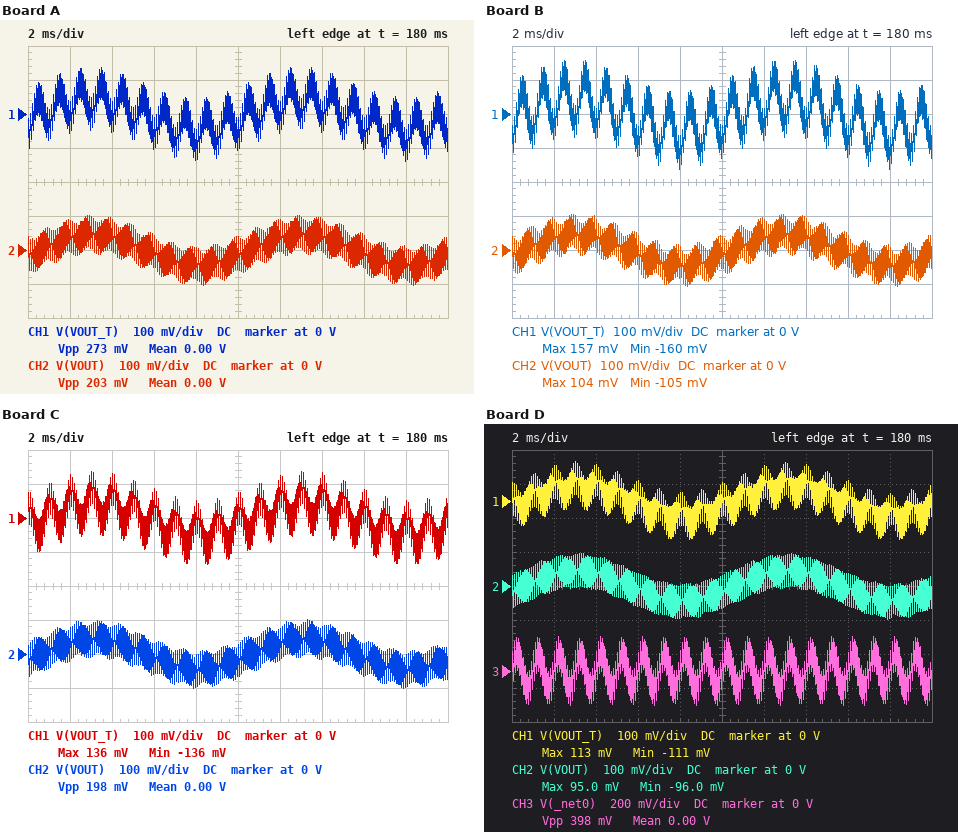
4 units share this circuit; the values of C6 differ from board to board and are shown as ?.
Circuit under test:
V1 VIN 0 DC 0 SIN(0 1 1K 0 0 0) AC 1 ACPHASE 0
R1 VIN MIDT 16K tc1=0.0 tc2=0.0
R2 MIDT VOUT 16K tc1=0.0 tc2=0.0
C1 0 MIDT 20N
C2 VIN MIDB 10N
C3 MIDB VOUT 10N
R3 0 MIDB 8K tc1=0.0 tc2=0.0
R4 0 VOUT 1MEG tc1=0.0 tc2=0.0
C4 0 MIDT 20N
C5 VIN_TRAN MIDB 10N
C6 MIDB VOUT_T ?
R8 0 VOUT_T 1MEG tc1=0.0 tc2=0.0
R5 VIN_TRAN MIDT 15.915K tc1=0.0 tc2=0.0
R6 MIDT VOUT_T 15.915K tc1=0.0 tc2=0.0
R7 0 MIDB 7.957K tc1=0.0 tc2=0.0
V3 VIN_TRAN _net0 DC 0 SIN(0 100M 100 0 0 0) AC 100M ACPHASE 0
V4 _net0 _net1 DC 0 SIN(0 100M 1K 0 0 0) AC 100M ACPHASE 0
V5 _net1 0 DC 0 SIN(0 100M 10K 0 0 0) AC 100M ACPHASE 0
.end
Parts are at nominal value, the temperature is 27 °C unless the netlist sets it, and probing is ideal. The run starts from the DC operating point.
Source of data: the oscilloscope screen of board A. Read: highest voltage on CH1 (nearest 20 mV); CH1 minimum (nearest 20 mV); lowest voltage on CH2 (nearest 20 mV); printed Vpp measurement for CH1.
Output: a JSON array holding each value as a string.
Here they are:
["140 mV", "-140 mV", "-100 mV", "273 mV"]
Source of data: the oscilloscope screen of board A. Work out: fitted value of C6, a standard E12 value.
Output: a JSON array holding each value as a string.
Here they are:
["6.8 nF"]
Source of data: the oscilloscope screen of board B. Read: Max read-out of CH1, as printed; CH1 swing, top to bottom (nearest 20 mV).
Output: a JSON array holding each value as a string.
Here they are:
["157 mV", "320 mV"]
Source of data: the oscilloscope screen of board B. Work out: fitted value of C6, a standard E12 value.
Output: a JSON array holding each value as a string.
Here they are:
["5.6 nF"]
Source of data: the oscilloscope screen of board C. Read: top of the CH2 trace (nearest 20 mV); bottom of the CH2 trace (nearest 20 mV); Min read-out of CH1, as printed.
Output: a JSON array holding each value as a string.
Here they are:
["100 mV", "-100 mV", "-136 mV"]
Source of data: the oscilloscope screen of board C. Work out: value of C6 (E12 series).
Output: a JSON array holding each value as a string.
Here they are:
["15 nF"]
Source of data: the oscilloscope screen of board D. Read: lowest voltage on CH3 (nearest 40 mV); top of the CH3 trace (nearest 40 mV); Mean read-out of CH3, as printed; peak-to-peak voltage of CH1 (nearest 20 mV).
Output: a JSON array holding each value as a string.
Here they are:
["-200 mV", "200 mV", "0.00 V", "220 mV"]
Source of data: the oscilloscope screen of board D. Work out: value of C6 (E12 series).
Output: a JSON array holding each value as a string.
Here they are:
["12 nF"]
